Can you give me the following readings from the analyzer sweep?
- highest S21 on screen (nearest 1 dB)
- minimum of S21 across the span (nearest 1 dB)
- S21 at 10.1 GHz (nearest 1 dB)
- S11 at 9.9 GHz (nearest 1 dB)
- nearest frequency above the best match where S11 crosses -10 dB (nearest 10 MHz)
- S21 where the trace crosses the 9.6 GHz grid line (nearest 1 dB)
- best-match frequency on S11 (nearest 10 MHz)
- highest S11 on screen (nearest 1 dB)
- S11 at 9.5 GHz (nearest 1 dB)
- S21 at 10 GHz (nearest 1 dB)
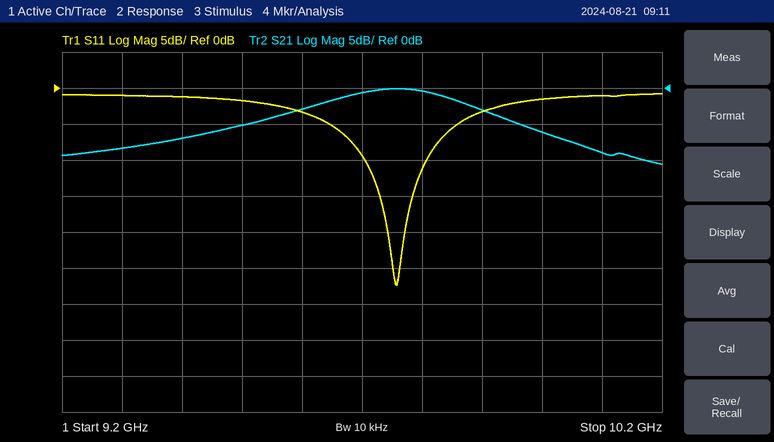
0 dB
-11 dB
-9 dB
-3 dB
9.81 GHz
-3 dB
9.76 GHz
-1 dB
-2 dB
-6 dB
